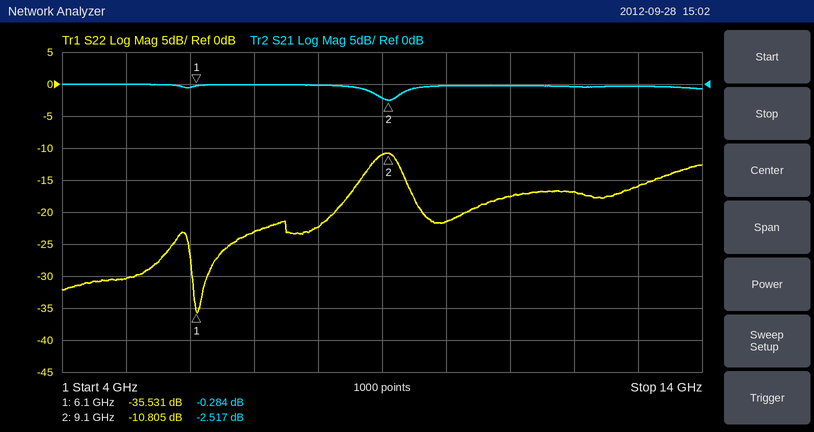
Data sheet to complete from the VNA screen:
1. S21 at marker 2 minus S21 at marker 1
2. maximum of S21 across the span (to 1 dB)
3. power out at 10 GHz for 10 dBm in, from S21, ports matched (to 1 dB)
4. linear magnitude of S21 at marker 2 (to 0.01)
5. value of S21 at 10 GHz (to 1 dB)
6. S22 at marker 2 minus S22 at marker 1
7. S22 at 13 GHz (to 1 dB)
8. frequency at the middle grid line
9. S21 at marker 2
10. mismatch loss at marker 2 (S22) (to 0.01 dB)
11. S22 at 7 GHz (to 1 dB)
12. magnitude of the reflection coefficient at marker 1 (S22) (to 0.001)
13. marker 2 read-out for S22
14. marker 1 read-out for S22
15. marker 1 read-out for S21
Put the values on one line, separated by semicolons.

-2.233 dB; 0 dB; 10 dBm; 0.75; 0 dB; 24.726 dB; -16 dB; 9 GHz; -2.517 dB; 0.38 dB; -23 dB; 0.017; -10.805 dB; -35.531 dB; -0.284 dB
